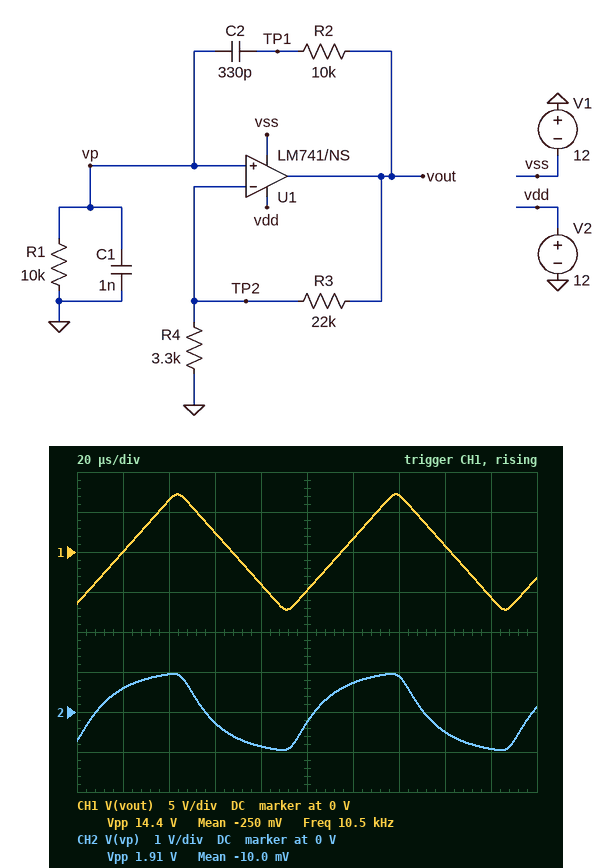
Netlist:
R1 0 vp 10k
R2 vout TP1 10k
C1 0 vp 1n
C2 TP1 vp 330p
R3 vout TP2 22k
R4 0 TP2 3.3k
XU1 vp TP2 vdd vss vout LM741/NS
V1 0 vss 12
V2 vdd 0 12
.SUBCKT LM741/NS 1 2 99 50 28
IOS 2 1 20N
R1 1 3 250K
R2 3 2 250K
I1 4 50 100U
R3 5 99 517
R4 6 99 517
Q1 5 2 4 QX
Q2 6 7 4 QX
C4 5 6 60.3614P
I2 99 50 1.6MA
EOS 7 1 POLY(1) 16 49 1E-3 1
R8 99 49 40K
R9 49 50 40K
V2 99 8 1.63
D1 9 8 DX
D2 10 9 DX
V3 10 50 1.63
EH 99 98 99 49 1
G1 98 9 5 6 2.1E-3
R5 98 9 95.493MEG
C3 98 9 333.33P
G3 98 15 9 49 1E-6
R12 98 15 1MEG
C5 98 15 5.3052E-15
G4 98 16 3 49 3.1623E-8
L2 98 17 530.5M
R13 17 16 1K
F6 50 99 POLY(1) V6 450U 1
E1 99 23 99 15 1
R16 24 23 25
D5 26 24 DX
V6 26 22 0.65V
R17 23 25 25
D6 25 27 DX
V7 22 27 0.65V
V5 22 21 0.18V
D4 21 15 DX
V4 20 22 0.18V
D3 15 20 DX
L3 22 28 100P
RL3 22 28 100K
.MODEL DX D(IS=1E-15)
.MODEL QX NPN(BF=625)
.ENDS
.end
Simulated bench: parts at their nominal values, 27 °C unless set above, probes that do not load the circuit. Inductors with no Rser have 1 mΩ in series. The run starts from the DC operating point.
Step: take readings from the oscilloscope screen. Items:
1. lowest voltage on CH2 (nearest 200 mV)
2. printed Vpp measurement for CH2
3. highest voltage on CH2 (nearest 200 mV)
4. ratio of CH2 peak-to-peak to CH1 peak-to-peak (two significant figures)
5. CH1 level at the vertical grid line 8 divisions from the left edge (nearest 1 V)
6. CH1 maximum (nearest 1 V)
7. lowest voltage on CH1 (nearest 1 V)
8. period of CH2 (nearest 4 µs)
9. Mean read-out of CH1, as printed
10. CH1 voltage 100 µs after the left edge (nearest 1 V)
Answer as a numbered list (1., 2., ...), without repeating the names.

1. -1.0 V
2. 1.91 V
3. 1.0 V
4. 0.13
5. 1 V
6. 7 V
7. -7 V
8. 96 µs
9. -250 mV
10. -5 V
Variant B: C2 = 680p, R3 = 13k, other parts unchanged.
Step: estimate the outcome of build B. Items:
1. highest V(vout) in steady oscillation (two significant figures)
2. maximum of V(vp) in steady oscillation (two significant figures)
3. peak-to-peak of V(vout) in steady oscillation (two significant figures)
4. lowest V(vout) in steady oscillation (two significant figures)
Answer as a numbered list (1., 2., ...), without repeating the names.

1. 9.5 V
2. 1.9 V
3. 19 V
4. -9.5 V
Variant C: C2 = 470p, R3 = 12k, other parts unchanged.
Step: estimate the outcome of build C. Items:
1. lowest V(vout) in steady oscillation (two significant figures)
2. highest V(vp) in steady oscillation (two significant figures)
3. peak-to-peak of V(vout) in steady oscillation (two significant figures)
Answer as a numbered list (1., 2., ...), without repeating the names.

1. -4.7 V
2. 1.0 V
3. 9.5 V
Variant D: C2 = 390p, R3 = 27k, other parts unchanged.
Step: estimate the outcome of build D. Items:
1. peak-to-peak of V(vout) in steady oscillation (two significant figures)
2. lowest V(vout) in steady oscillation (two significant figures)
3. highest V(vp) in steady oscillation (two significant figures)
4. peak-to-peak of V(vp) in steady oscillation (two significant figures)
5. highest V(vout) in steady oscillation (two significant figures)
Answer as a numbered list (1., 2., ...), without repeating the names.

1. 22 V
2. -11 V
3. 1.2 V
4. 2.4 V
5. 11 V
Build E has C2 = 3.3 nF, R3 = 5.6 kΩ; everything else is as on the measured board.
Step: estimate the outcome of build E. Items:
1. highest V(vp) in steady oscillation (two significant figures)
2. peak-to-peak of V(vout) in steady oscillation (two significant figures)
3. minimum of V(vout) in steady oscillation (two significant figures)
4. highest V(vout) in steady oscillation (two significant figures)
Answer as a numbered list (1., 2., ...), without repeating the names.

1. 4.8 V
2. 22 V
3. -11 V
4. 11 V
